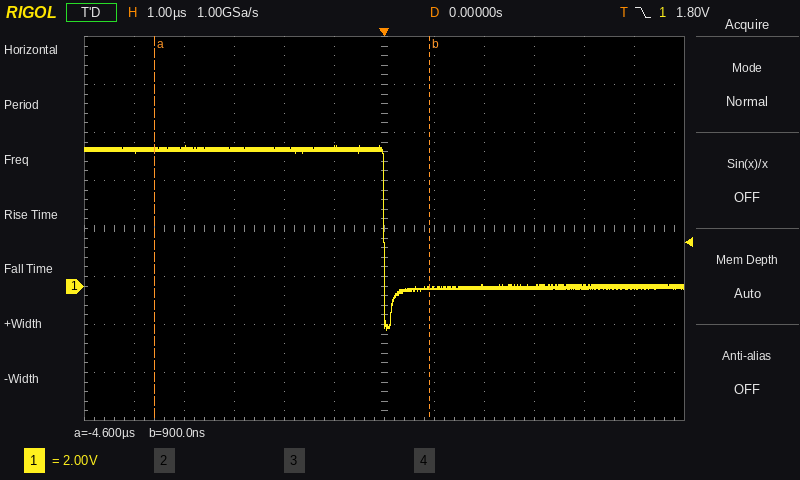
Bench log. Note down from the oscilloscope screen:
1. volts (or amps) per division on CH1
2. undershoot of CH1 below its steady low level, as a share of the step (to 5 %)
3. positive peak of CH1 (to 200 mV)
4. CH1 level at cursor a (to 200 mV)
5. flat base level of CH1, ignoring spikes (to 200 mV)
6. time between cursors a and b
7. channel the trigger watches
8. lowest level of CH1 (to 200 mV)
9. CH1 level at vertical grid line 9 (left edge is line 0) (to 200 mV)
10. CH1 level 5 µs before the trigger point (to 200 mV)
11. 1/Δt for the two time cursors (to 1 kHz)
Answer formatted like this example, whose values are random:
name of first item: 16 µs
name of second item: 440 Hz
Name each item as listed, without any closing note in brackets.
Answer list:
volts (or amps) per division on CH1: 2 V
undershoot of CH1 below its steady low level, as a share of the step: 30 %
positive peak of CH1: 5.8 V
CH1 level at cursor a: 5.6 V
flat base level of CH1, ignoring spikes: 0.0 V
time between cursors a and b: 5.5 µs
channel the trigger watches: CH1
lowest level of CH1: -1.8 V
CH1 level at vertical grid line 9 (left edge is line 0): 0.0 V
CH1 level 5 µs before the trigger point: 5.6 V
1/Δt for the two time cursors: 182 kHz
